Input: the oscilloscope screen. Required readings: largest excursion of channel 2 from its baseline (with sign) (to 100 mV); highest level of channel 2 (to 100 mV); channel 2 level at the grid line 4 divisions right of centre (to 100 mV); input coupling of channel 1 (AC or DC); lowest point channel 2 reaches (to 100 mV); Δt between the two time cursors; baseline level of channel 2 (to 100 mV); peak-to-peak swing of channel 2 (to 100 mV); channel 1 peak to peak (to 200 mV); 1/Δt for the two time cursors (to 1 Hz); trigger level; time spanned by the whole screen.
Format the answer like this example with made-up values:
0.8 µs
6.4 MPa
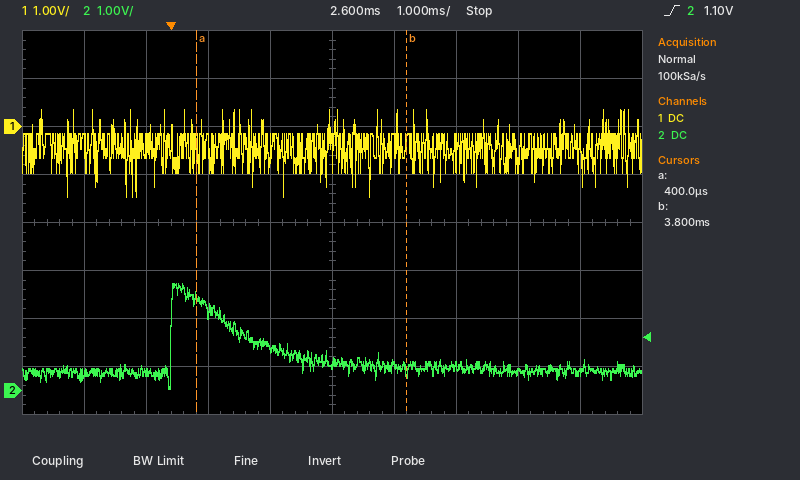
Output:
+1.8 V
2.2 V
400 mV
DC
0.0 V
3.4 ms
400 mV
2.2 V
1.8 V
294 Hz
1.10 V
10 ms
